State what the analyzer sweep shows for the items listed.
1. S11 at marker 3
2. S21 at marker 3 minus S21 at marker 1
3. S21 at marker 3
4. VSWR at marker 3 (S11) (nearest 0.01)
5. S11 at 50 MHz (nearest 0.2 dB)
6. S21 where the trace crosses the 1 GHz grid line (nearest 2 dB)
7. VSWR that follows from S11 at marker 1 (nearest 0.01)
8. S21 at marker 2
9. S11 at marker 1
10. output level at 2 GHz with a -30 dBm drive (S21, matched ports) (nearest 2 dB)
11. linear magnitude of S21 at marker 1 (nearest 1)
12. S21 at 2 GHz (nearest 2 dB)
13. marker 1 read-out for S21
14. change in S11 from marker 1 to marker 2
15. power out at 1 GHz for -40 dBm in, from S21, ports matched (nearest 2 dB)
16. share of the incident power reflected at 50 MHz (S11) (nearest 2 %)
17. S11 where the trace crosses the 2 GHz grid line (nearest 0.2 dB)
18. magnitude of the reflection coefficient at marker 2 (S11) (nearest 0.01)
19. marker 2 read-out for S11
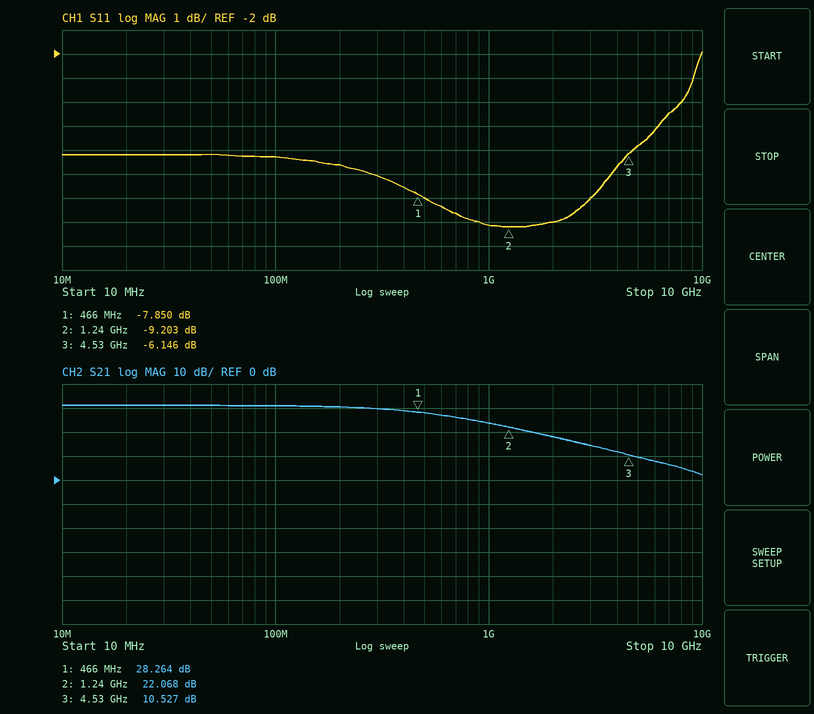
-6.146 dB
-17.737 dB
10.527 dB
2.94
-6.2 dB
24 dB
2.36
22.068 dB
-7.850 dB
-12 dBm
26
18 dB
28.264 dB
-1.353 dB
-16 dBm
24 %
-9.0 dB
0.35
-9.203 dB
